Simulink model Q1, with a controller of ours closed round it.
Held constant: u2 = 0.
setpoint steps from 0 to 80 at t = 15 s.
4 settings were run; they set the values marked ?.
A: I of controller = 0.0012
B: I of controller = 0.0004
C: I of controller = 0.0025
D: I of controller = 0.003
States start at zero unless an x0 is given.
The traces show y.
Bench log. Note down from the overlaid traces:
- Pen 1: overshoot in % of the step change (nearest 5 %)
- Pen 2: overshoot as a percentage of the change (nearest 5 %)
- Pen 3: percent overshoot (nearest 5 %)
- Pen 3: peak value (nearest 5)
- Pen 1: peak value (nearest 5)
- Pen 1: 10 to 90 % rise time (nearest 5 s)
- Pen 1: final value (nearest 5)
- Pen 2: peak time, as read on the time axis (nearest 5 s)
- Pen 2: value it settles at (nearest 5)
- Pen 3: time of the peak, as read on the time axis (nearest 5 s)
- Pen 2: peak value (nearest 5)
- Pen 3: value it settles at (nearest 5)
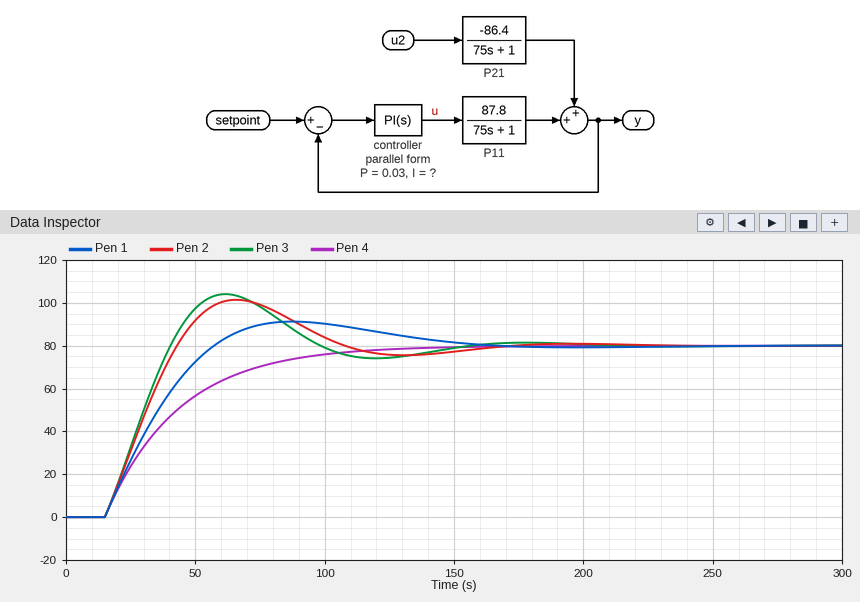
15 %
25 %
30 %
105
90
30 s
80
65 s
80
60 s
100
80
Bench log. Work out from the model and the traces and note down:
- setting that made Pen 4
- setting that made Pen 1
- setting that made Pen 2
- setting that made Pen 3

B
A
C
D
